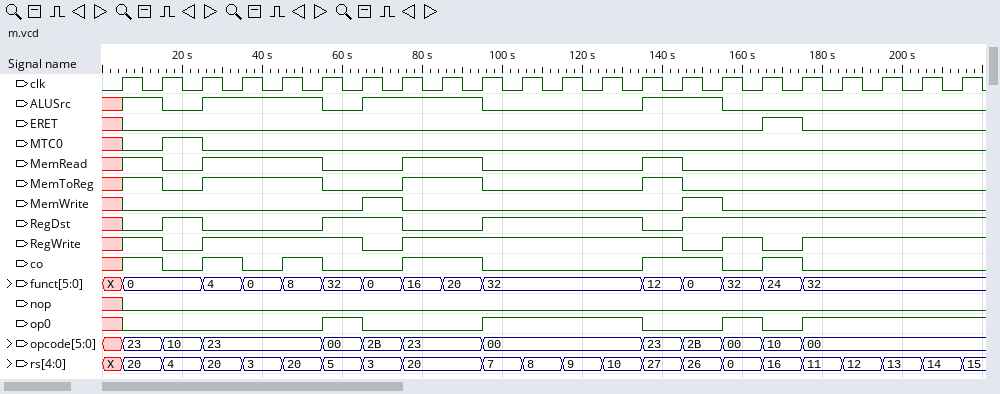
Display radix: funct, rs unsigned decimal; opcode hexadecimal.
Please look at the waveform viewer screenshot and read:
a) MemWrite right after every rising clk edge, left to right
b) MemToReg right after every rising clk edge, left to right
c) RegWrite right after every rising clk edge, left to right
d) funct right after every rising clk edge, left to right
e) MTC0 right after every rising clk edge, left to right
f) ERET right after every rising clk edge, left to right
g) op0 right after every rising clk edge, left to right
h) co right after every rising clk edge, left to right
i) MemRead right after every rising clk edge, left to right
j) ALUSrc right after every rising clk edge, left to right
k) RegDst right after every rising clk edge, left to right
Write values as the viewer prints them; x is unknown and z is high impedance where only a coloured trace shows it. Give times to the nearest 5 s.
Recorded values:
0 0 0 0 0 0 1 0 0 0 0 0 0 0 1 0 0 0 0 0 0 0
1 0 1 1 1 0 0 1 1 0 0 0 0 1 0 0 0 0 0 0 0 0
1 0 1 1 1 1 0 1 1 1 1 1 1 1 0 1 0 1 1 1 1 1
0, 0, 4, 0, 8, 32, 0, 16, 20, 32, 32, 32, 32, 12, 0, 32, 24, 32, 32, 32, 32, 32
0 1 0 0 0 0 0 0 0 0 0 0 0 0 0 0 0 0 0 0 0 0
0 0 0 0 0 0 0 0 0 0 0 0 0 0 0 0 1 0 0 0 0 0
0 0 0 0 0 1 0 0 0 1 1 1 1 0 0 1 0 1 1 1 1 1
1 0 1 0 1 0 0 1 1 0 0 0 0 1 1 0 1 0 0 0 0 0
1 0 1 1 1 0 0 1 1 0 0 0 0 1 0 0 0 0 0 0 0 0
1 0 1 1 1 0 1 1 1 0 0 0 0 1 1 0 0 0 0 0 0 0
0 1 0 0 0 1 1 0 0 1 1 1 1 0 1 1 1 1 1 1 1 1
